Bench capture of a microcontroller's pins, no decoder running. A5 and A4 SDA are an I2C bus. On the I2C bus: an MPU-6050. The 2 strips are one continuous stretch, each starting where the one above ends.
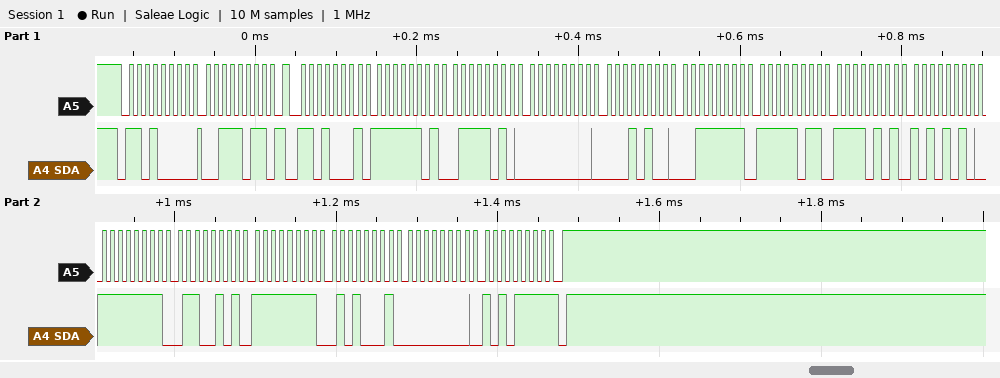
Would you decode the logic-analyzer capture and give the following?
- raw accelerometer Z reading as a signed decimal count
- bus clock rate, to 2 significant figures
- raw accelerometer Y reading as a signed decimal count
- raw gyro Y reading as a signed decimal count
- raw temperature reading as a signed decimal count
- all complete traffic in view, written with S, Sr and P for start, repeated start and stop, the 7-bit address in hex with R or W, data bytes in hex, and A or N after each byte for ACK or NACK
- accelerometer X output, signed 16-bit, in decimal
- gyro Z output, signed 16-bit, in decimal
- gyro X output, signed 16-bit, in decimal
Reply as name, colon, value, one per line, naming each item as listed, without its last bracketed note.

raw accelerometer Z reading as a signed decimal count: 16379
bus clock rate, to 2 significant figures: 100 kHz
raw accelerometer Y reading as a signed decimal count: 20
raw gyro Y reading as a signed decimal count: -175
raw temperature reading as a signed decimal count: -2646
all complete traffic in view, written with S, Sr and P for start, repeated start and stop, the 7-bit address in hex with R or W, data bytes in hex, and A or N after each byte for ACK or NACK: S 68W A 3B A Sr 68R A FD A 7A A 00 A 14 A 3F A FB A F5 A AA A FF A 65 A FF A 51 A 00 A AF N P
accelerometer X output, signed 16-bit, in decimal: -646
gyro Z output, signed 16-bit, in decimal: 175
gyro X output, signed 16-bit, in decimal: -155
